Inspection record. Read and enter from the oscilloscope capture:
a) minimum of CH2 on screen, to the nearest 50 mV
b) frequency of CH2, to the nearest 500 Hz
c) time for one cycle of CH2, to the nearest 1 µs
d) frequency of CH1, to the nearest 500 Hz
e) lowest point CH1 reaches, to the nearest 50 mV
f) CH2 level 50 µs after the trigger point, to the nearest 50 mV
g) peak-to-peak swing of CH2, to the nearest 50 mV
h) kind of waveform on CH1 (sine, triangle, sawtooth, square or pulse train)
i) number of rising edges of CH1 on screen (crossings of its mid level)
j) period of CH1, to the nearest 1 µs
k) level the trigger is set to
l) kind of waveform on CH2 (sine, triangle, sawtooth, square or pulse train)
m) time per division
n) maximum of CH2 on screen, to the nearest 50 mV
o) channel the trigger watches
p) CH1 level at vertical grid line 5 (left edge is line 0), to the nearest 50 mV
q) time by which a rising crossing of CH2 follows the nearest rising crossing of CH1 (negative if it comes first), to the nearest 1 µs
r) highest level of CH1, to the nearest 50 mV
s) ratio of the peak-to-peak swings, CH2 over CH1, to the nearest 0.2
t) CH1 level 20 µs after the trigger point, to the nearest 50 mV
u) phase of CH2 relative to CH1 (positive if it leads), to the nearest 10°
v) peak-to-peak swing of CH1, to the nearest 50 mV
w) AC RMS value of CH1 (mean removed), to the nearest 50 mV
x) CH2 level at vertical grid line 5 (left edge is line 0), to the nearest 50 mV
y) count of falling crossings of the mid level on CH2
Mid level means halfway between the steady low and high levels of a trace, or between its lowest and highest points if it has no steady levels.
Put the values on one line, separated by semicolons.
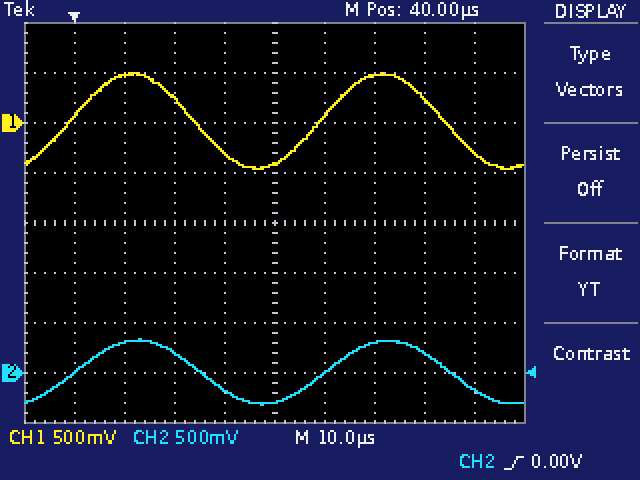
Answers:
-300 mV; 20.0 kHz; 50 µs; 20.0 kHz; -450 mV; 0 mV; 650 mV; sine; 2; 50 µs; 0.00 V; sine; 10 µs; 350 mV; CH2; -400 mV; +1 µs; 500 mV; 0.6; 250 mV; -10°; 950 mV; 350 mV; -300 mV; 2
